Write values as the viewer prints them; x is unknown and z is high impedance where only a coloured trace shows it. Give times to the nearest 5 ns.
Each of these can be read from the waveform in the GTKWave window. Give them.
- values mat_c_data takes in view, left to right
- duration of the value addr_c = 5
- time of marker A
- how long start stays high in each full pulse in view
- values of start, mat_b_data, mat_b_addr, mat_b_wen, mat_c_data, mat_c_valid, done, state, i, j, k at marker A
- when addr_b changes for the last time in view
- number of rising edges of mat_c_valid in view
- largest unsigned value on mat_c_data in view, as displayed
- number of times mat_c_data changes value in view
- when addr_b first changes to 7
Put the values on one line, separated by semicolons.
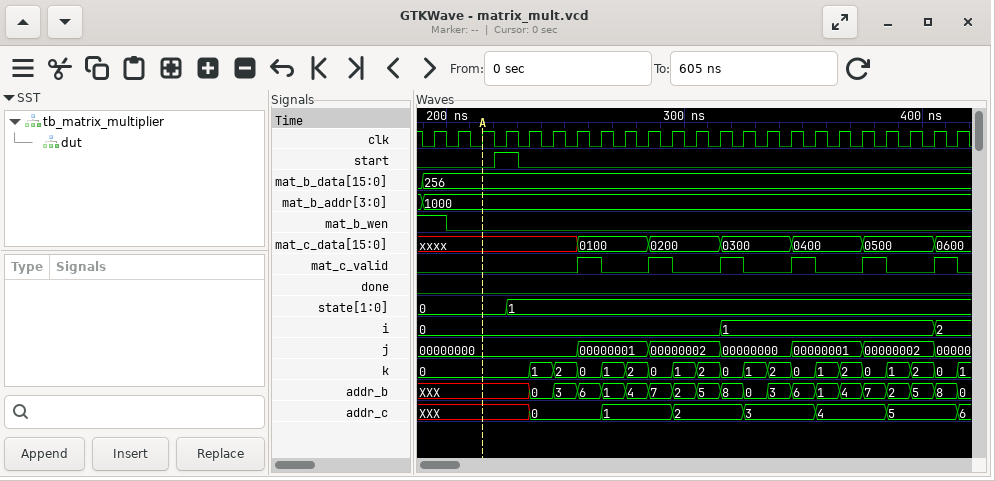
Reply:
xxxx, 0100, 0200, 0300, 0400, 0500, 0600; 30 ns; 215 ns; 10 ns; start=0, mat_b_data=256, mat_b_addr=1000, mat_b_wen=0, mat_c_data=xxxx, mat_c_valid=0, done=0, state=0, i=0, j=00000000, k=0; 415 ns; 6; 0600; 6; 285 ns
